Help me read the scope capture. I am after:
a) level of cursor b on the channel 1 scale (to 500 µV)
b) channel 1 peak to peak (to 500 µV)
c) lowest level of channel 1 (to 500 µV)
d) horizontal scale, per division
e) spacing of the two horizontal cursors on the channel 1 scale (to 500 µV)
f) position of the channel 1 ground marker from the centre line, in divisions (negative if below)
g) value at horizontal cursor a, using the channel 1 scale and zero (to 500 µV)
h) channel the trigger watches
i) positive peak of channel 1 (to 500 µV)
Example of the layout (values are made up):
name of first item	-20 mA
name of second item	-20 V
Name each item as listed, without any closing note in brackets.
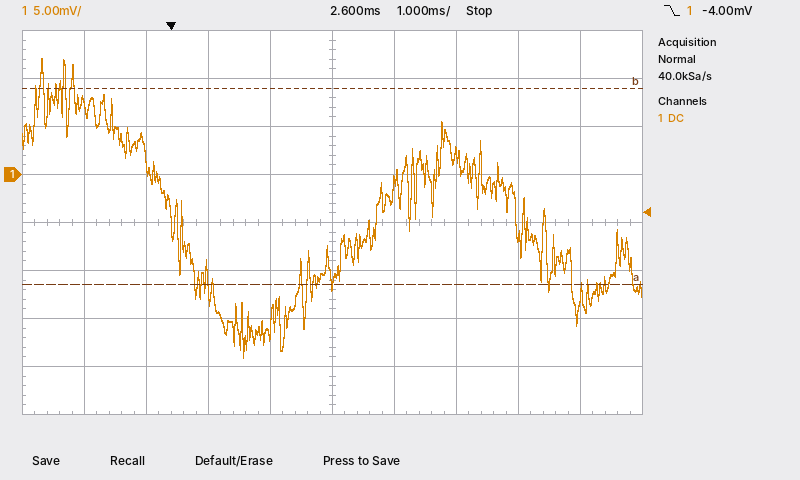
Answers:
level of cursor b on the channel 1 scale	9.0 mV
channel 1 peak to peak	31.0 mV
lowest level of channel 1	-19.0 mV
horizontal scale, per division	1 ms
spacing of the two horizontal cursors on the channel 1 scale	20.5 mV
position of the channel 1 ground marker from the centre line, in divisions	+1.0 div
value at horizontal cursor a, using the channel 1 scale and zero	-11.5 mV
channel the trigger watches	channel 1
positive peak of channel 1	12.0 mV
